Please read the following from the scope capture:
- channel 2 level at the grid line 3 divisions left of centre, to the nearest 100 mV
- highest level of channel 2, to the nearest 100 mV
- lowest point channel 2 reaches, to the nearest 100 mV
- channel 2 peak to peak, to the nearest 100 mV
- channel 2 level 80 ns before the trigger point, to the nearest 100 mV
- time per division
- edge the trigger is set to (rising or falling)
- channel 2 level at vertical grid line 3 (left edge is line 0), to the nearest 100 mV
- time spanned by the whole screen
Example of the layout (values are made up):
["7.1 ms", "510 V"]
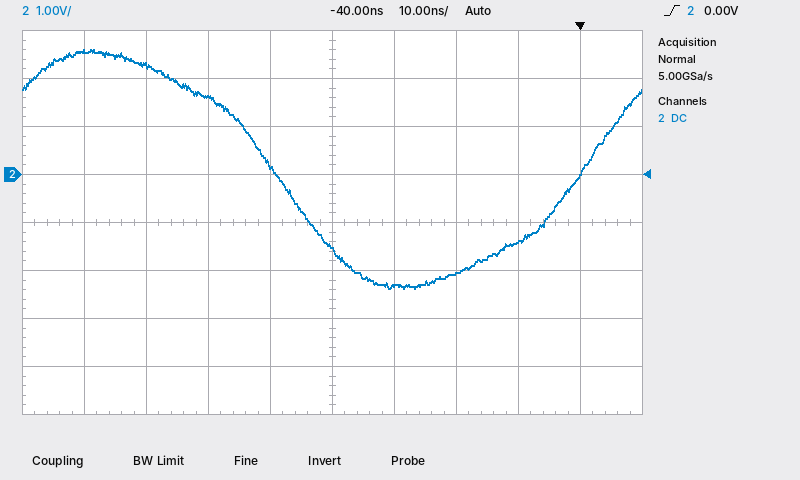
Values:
["2.3 V", "2.6 V", "-2.4 V", "5.0 V", "2.6 V", "10 ns", "rising", "1.6 V", "100 ns"]
